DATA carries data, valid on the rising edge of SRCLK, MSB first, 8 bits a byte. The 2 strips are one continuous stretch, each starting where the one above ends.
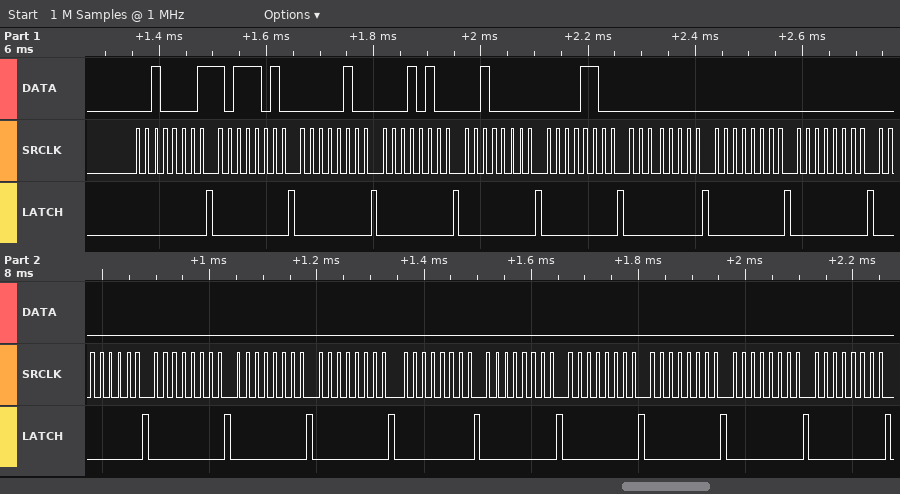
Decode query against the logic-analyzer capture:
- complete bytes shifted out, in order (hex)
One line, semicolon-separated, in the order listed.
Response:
0x21 0xBA 0x04 0x14 0x20 0x0C 0x00 0x00 0x00 0x00 0x00 0x00 0x00 0x00 0x00 0x00 0x00 0x00 0x00
